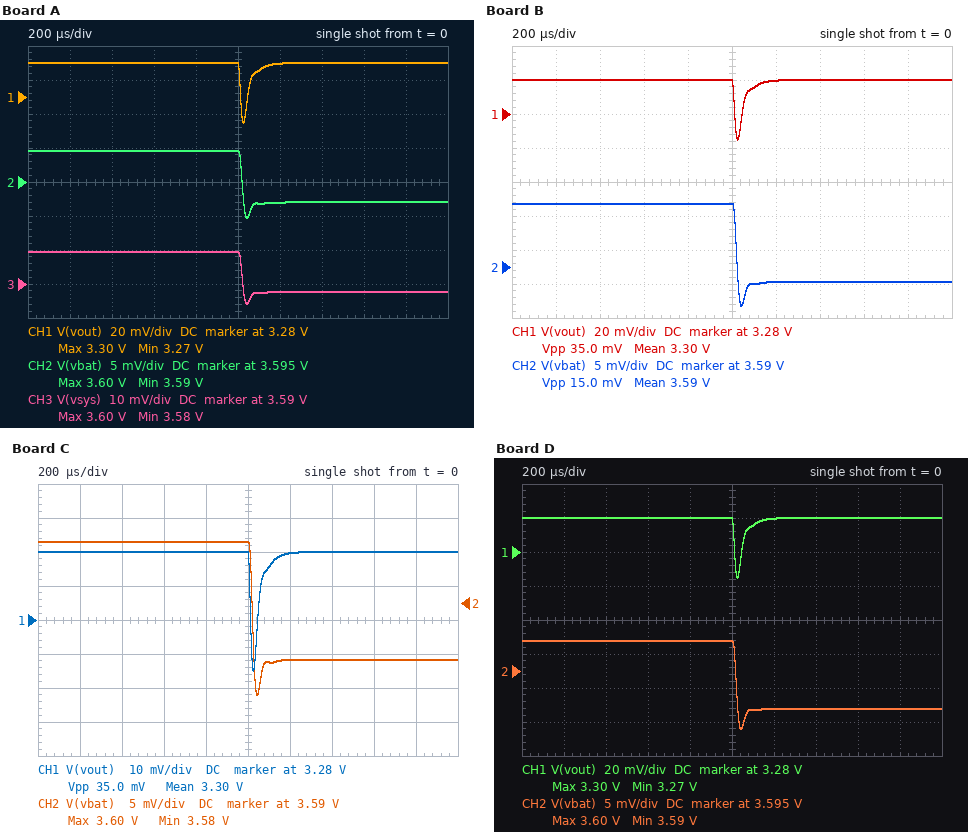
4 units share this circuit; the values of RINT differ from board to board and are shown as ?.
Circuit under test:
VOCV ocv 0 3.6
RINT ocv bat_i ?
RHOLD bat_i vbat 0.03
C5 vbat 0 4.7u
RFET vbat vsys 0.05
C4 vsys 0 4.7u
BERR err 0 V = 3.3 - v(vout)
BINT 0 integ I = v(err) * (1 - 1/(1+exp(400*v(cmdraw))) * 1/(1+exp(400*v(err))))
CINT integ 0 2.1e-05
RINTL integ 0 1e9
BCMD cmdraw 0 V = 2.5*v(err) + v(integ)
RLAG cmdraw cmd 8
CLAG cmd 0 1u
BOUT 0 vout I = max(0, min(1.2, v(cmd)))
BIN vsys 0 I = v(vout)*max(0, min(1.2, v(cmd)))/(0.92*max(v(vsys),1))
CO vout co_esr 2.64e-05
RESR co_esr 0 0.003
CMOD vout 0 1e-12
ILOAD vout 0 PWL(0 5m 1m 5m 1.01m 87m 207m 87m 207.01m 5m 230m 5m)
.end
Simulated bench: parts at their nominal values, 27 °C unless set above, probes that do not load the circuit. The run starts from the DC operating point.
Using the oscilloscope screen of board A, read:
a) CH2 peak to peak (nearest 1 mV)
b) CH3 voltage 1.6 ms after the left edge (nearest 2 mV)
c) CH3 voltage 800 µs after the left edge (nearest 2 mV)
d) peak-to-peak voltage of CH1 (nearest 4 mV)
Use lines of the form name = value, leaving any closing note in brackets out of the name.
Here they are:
CH2 peak to peak = 10 mV
CH3 voltage 1.6 ms after the left edge = 3.588 V
CH3 voltage 800 µs after the left edge = 3.600 V
peak-to-peak voltage of CH1 = 36 mV
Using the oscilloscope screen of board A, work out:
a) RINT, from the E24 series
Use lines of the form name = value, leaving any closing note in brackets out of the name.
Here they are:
RINT, from the E24 series = 0.062 Ω
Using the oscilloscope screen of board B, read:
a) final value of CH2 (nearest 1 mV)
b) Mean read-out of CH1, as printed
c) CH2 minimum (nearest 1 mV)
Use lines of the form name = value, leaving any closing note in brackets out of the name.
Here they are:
final value of CH2 = 3.588 V
Mean read-out of CH1, as printed = 3.30 V
CH2 minimum = 3.584 V
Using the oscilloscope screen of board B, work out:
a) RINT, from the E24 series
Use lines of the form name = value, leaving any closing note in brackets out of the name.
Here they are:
RINT, from the E24 series = 0.11 Ω
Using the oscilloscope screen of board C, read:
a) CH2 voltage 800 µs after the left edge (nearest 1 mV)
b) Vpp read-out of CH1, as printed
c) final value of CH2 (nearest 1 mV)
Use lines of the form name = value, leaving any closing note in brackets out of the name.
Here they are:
CH2 voltage 800 µs after the left edge = 3.599 V
Vpp read-out of CH1, as printed = 35.0 mV
final value of CH2 = 3.582 V
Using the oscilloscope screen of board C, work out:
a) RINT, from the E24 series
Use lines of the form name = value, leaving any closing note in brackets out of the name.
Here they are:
RINT, from the E24 series = 0.18 Ω
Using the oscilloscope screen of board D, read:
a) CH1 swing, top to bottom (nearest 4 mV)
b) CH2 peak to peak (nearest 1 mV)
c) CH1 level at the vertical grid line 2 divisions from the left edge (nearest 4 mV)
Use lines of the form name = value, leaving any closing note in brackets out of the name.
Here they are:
CH1 swing, top to bottom = 36 mV
CH2 peak to peak = 13 mV
CH1 level at the vertical grid line 2 divisions from the left edge = 3.300 V
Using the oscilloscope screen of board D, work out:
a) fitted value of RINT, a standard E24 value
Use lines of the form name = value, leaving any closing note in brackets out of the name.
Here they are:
fitted value of RINT, a standard E24 value = 0.091 Ω
